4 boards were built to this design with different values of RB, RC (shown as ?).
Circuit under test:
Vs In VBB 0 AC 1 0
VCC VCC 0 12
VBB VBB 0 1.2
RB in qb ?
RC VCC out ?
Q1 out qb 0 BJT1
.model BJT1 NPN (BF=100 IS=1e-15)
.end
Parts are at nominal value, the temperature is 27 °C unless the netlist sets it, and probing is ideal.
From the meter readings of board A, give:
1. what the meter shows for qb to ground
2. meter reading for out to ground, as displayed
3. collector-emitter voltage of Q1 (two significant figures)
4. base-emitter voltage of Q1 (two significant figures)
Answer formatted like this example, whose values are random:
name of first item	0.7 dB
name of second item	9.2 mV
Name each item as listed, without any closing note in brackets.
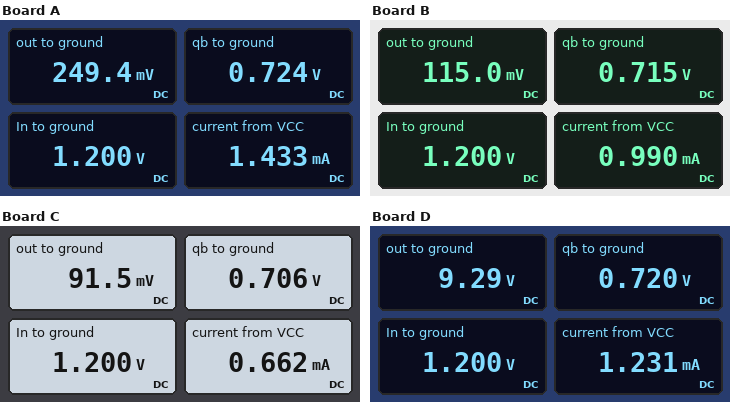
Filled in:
what the meter shows for qb to ground	0.724 V
meter reading for out to ground, as displayed	249.4 mV
collector-emitter voltage of Q1	250 mV
base-emitter voltage of Q1	720 mV
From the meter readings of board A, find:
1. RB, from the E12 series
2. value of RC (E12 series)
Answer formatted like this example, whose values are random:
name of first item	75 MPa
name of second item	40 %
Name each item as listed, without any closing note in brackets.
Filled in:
RB, from the E12 series	33 kΩ
value of RC	8.2 kΩ
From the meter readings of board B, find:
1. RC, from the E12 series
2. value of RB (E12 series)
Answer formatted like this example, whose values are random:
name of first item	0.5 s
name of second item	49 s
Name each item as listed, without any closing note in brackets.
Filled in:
RC, from the E12 series	12 kΩ
value of RB	22 kΩ
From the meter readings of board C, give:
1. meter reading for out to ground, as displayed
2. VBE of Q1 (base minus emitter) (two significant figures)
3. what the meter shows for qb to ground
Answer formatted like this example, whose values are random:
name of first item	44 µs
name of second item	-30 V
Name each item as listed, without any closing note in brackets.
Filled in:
meter reading for out to ground, as displayed	91.5 mV
VBE of Q1 (base minus emitter)	710 mV
what the meter shows for qb to ground	0.706 V
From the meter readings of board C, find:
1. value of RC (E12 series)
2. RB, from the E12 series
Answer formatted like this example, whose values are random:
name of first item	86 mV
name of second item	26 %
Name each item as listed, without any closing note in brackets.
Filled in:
value of RC	18 kΩ
RB, from the E12 series	18 kΩ
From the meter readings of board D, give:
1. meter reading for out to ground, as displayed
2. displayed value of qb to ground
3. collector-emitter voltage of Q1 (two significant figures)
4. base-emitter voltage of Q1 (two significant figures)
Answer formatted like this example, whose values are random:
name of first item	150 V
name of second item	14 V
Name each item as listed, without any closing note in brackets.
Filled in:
meter reading for out to ground, as displayed	9.29 V
displayed value of qb to ground	0.720 V
collector-emitter voltage of Q1	9.3 V
base-emitter voltage of Q1	720 mV
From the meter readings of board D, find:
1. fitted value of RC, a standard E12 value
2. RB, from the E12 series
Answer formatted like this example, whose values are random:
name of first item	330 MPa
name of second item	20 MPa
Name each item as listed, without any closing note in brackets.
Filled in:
fitted value of RC, a standard E12 value	2.2 kΩ
RB, from the E12 series	39 kΩ
